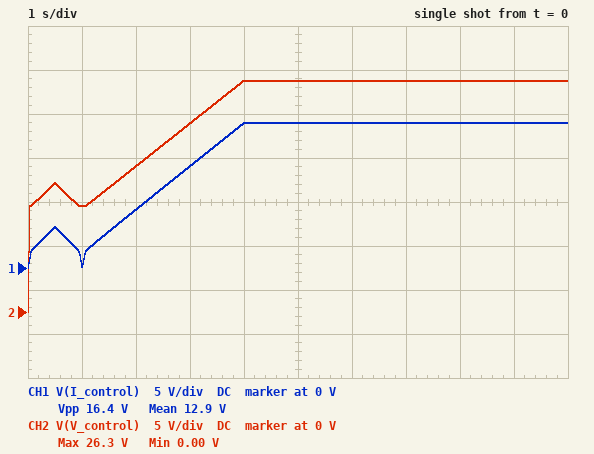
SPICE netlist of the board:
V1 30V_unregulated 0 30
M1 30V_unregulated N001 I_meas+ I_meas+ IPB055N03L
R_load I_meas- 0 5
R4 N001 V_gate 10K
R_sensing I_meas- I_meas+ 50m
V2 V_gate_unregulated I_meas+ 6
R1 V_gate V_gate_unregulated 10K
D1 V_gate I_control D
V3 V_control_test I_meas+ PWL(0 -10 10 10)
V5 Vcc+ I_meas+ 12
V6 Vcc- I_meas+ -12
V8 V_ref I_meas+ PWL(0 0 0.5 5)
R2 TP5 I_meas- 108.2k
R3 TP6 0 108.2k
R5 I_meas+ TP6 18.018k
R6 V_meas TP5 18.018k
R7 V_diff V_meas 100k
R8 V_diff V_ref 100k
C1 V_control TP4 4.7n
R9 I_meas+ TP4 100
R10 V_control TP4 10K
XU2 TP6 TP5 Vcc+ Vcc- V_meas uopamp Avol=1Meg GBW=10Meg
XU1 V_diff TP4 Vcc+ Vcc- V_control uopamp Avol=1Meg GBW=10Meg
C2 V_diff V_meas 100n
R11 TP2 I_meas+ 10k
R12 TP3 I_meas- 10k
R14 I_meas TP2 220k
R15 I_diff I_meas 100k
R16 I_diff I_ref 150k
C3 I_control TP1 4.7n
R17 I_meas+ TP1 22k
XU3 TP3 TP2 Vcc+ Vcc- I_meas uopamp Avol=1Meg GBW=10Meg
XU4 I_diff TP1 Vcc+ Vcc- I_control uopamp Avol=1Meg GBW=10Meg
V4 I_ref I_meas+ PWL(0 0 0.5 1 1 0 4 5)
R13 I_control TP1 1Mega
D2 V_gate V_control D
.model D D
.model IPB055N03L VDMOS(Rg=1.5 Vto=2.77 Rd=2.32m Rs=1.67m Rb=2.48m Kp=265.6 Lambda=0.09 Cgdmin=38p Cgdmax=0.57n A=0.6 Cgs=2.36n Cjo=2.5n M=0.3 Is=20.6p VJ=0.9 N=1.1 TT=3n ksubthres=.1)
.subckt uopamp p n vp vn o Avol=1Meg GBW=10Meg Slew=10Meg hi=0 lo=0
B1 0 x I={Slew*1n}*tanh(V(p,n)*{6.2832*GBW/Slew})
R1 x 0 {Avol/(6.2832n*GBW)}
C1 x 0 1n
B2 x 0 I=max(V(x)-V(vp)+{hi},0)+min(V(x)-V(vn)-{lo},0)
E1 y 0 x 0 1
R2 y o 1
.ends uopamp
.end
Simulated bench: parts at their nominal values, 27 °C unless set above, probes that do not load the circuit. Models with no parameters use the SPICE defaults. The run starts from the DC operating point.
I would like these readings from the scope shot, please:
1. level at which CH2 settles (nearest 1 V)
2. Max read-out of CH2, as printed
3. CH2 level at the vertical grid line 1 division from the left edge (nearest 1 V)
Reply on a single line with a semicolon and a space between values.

26 V; 26.3 V; 12 V
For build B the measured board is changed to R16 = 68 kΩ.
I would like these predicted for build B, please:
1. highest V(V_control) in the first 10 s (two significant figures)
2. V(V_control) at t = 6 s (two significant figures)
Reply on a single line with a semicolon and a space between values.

41 V; 33 V
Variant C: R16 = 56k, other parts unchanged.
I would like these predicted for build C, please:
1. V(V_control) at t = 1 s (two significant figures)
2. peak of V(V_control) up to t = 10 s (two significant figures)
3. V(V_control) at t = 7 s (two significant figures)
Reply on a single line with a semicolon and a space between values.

12 V; 41 V; 33 V
